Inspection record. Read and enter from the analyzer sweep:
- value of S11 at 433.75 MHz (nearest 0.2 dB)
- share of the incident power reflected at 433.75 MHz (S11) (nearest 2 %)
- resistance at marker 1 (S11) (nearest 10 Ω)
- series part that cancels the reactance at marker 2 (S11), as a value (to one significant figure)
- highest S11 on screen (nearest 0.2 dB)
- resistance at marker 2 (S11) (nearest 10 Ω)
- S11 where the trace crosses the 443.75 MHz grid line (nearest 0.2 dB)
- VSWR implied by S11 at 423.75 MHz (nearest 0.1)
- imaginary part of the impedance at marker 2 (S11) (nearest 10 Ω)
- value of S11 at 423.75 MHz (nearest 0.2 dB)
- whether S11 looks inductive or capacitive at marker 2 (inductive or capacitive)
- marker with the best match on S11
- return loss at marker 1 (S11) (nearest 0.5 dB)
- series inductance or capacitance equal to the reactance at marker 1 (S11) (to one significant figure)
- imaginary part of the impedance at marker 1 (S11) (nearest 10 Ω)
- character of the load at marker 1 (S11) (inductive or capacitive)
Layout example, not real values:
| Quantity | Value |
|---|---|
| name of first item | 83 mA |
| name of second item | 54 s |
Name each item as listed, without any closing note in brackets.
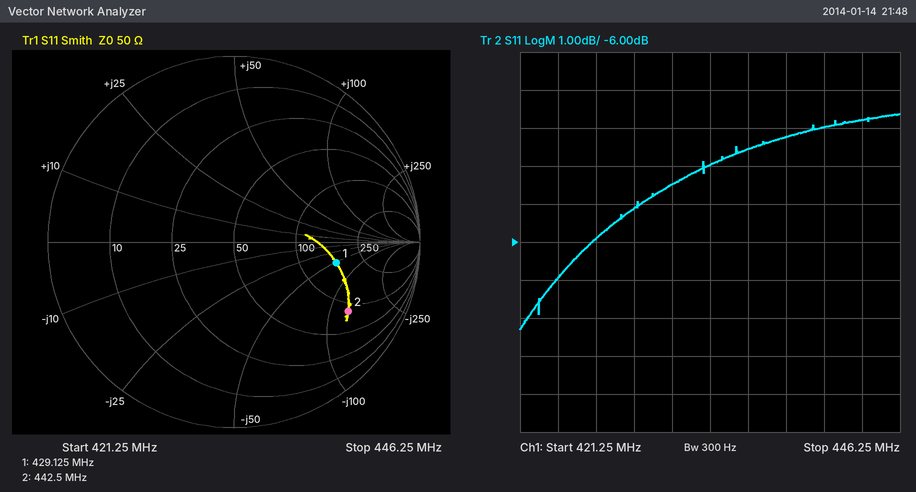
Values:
| Quantity | Value |
|---|---|
| value of S11 at 433.75 MHz | -4.0 dB |
| share of the incident power reflected at 433.75 MHz (S11) | 40 % |
| resistance at marker 1 (S11) | 160 Ω |
| series part that cancels the reactance at marker 2 (S11), as a value | 50 nH |
| highest S11 on screen | -2.6 dB |
| resistance at marker 2 (S11) | 80 Ω |
| S11 where the trace crosses the 443.75 MHz grid line | -2.8 dB |
| VSWR implied by S11 at 423.75 MHz | 2.6 |
| imaginary part of the impedance at marker 2 (S11) | -130 Ω |
| value of S11 at 423.75 MHz | -7.0 dB |
| whether S11 looks inductive or capacitive at marker 2 | capacitive |
| marker with the best match on S11 | marker 1 |
| return loss at marker 1 (S11) | 5.0 dB |
| series inductance or capacitance equal to the reactance at marker 1 (S11) | 7 pF |
| imaginary part of the impedance at marker 1 (S11) | -50 Ω |
| character of the load at marker 1 (S11) | capacitive |
